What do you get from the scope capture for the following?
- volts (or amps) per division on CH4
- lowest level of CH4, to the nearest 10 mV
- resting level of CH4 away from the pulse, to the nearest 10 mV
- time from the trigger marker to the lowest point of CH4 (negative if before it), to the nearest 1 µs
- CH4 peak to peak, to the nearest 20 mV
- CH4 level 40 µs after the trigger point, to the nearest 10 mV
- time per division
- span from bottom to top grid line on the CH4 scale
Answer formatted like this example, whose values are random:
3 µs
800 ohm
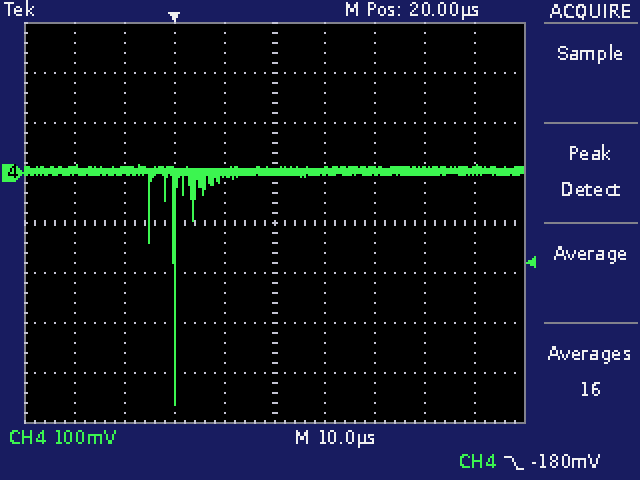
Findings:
100 mV
-460 mV
0 mV
0 µs
480 mV
0 mV
10 µs
800 mV
